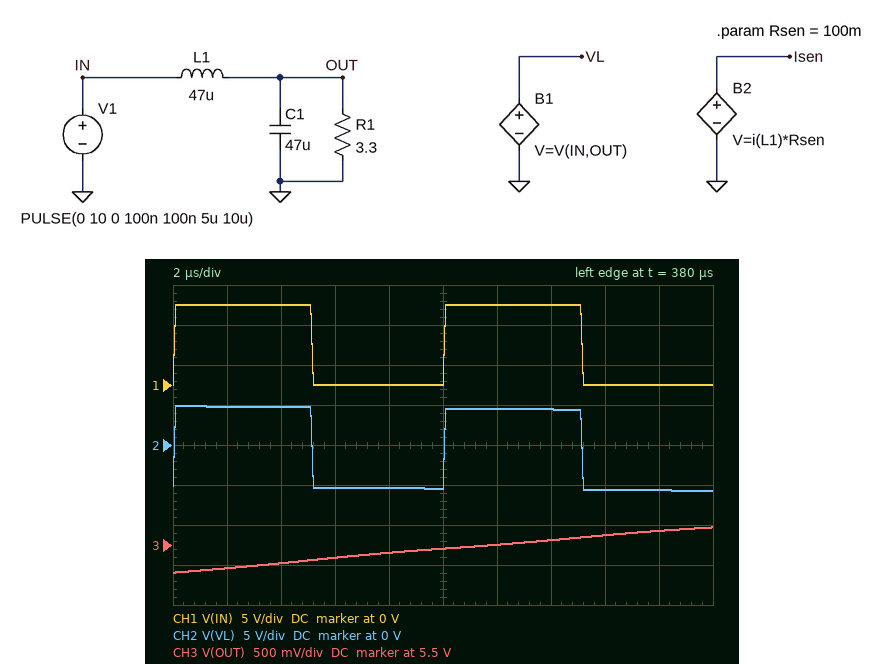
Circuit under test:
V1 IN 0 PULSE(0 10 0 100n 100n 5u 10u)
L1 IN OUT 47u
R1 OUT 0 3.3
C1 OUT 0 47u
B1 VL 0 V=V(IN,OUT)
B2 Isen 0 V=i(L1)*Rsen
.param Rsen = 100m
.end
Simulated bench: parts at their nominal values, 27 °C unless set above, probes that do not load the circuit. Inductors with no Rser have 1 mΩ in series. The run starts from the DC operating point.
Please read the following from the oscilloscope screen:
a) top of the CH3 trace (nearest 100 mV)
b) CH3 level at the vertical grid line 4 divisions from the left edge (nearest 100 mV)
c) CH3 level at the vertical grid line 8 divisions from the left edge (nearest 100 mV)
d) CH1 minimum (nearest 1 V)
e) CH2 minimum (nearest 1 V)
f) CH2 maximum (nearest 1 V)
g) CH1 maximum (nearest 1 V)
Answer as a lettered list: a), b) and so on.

a) 5.7 V
b) 5.4 V
c) 5.6 V
d) 0 V
e) -6 V
f) 5 V
g) 10 V
